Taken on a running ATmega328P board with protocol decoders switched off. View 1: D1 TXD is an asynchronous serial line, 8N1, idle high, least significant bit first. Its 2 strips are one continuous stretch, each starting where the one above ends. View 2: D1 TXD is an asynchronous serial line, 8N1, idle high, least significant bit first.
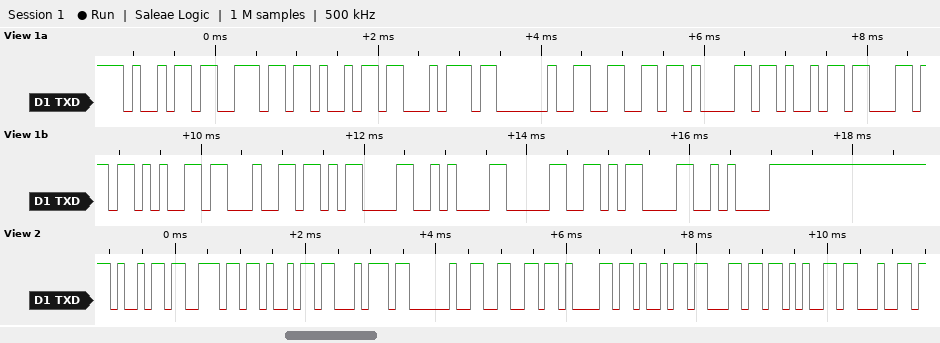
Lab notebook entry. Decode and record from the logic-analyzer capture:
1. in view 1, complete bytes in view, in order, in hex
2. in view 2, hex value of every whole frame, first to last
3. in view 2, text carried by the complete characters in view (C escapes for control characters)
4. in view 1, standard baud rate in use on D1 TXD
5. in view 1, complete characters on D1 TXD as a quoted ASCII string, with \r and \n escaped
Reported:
69 6E 69 74 20 66 61 69 6C 65 64 0D 0A 30 0D 0A
69 6E 69 74 20 66 61 69 6C 65 64
"init failed"
9600 baud
"init failed\r\n0\r\n"
